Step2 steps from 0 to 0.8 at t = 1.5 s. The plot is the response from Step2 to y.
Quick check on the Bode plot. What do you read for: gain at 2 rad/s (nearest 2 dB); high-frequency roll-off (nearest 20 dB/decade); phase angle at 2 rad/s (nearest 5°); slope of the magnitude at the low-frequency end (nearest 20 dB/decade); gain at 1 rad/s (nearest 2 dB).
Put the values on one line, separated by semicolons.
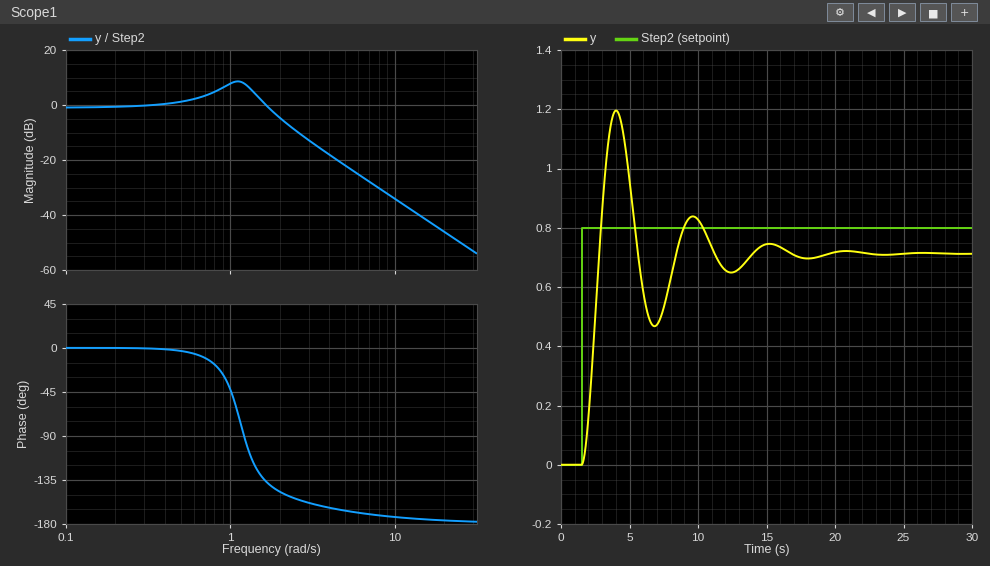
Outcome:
-4 dB; -40 dB/decade; -145°; 0 dB/decade; 8 dB
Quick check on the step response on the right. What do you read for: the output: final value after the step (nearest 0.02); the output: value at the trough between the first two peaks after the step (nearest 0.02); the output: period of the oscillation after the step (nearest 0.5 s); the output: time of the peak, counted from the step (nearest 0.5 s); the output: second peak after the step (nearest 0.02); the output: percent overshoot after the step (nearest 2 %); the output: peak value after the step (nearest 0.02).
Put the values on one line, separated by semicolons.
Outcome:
0.72; 0.46; 5.5 s; 2.5 s; 0.84; 68 %; 1.20
